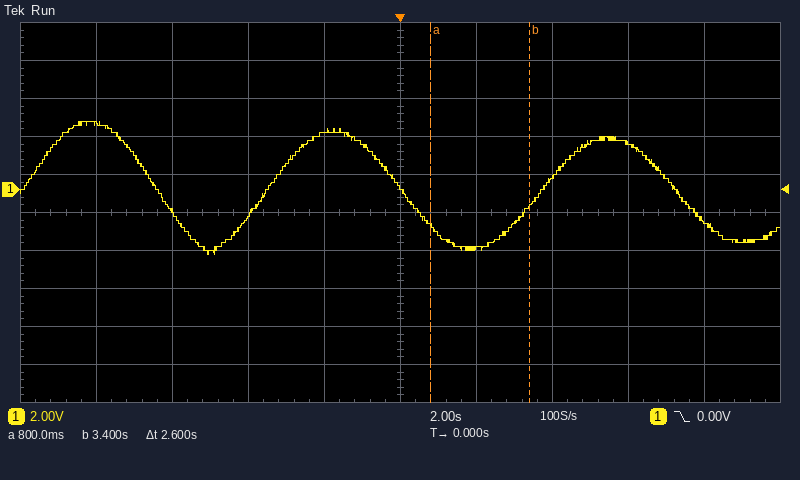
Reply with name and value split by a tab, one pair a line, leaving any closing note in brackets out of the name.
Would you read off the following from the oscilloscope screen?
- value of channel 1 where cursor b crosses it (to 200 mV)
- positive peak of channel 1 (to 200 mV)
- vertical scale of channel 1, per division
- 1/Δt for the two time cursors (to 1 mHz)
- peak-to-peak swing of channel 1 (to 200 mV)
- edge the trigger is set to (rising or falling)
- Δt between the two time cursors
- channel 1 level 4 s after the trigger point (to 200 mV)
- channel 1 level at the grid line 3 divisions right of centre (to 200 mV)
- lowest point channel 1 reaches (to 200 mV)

value of channel 1 where cursor b crosses it	-800 mV
positive peak of channel 1	3.6 V
vertical scale of channel 1, per division	2 V
1/Δt for the two time cursors	385 mHz
peak-to-peak swing of channel 1	7.0 V
edge the trigger is set to	falling
Δt between the two time cursors	2.6 s
channel 1 level 4 s after the trigger point	600 mV
channel 1 level at the grid line 3 divisions right of centre	2.4 V
lowest point channel 1 reaches	-3.4 V
